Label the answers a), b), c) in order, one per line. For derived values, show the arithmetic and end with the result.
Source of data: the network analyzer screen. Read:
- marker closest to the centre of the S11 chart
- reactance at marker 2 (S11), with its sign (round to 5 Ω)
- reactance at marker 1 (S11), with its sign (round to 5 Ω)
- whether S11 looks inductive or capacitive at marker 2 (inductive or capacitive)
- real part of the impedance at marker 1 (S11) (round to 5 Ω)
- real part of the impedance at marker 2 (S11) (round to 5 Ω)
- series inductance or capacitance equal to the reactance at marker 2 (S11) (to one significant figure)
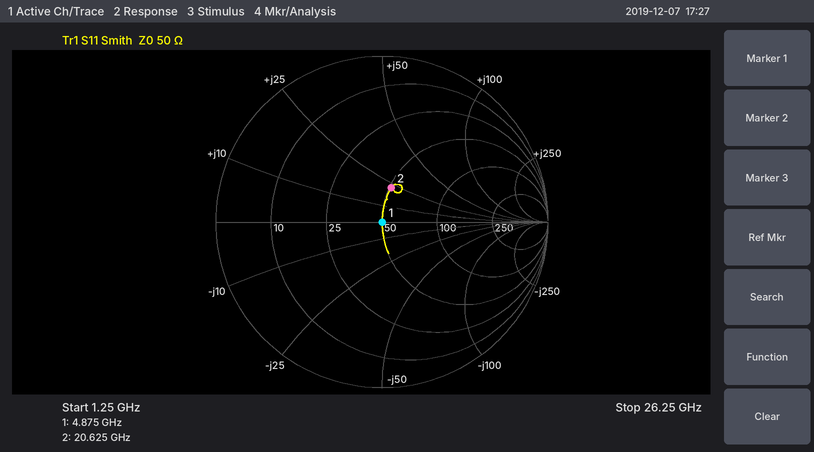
a) marker 1
b) +20 Ω
c) 0 Ω
d) inductive
e) 50 Ω
f) 50 Ω
g) L = 20 Ω/(2π × 20.625 GHz) ≈ 154 pH, so 200 pH to one significant figure
